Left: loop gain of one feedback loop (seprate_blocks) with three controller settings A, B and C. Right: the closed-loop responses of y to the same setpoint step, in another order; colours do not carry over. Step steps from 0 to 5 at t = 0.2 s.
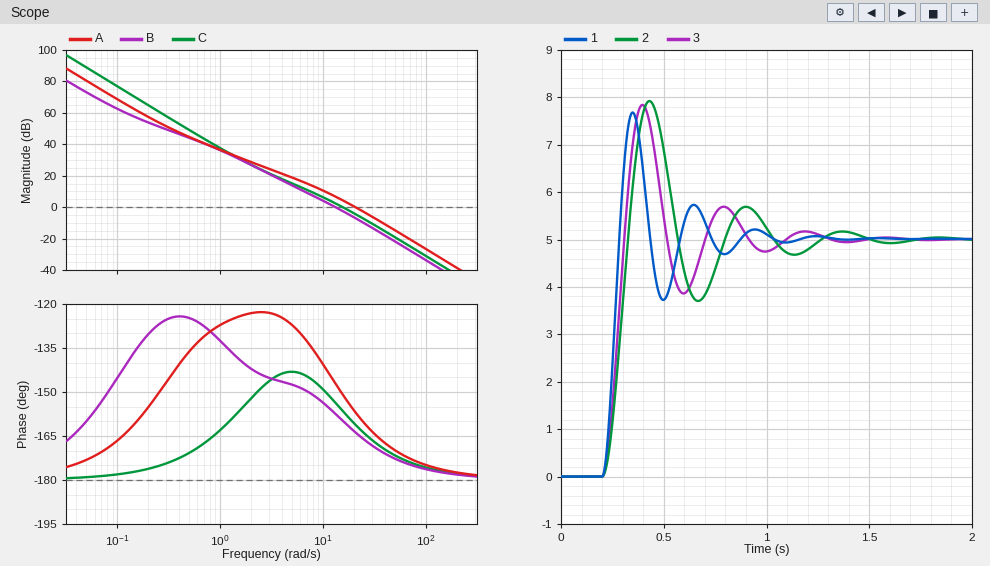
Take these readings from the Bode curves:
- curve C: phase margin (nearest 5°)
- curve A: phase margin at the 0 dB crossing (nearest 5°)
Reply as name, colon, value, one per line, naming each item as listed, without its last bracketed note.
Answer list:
curve C: phase margin: 25°
curve A: phase margin at the 0 dB crossing: 25°
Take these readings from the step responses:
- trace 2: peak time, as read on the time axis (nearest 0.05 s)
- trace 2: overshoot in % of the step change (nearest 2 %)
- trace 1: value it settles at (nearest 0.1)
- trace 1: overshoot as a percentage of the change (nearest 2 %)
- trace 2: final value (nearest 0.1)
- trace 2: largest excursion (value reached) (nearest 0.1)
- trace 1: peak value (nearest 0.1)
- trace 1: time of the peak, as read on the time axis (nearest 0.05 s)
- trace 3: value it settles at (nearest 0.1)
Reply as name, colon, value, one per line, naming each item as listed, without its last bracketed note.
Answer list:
trace 2: peak time, as read on the time axis: 0.45 s
trace 2: overshoot in % of the step change: 58 %
trace 1: value it settles at: 5.0
trace 1: overshoot as a percentage of the change: 54 %
trace 2: final value: 5.0
trace 2: largest excursion (value reached): 7.9
trace 1: peak value: 7.7
trace 1: time of the peak, as read on the time axis: 0.35 s
trace 3: value it settles at: 5.0
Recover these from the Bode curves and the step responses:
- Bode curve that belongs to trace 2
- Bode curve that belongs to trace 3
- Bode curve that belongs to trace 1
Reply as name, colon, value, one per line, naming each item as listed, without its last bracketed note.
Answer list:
Bode curve that belongs to trace 2: B
Bode curve that belongs to trace 3: C
Bode curve that belongs to trace 1: A
